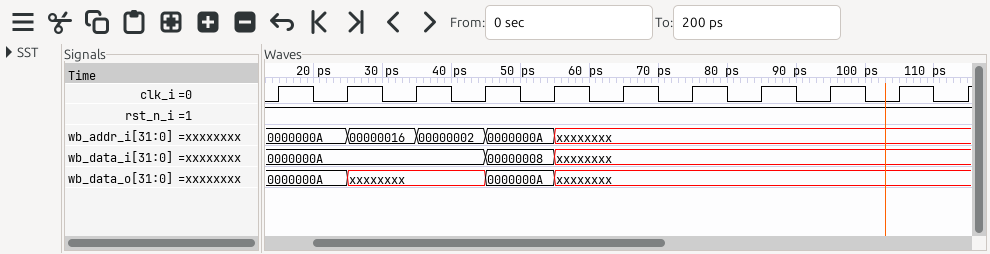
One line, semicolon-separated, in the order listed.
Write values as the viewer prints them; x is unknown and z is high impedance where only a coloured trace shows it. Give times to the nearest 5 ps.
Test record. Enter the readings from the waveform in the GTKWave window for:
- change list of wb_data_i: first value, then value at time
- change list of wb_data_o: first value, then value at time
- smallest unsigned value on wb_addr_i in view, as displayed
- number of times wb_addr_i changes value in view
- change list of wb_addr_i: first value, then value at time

0000000A, 00000008 at 45 ps, xxxxxxxx at 55 ps; 0000000A, xxxxxxxx at 25 ps, 0000000A at 45 ps, xxxxxxxx at 55 ps; 00000002; 4; 0000000A, 00000016 at 25 ps, 00000002 at 35 ps, 0000000A at 45 ps, xxxxxxxx at 55 ps
